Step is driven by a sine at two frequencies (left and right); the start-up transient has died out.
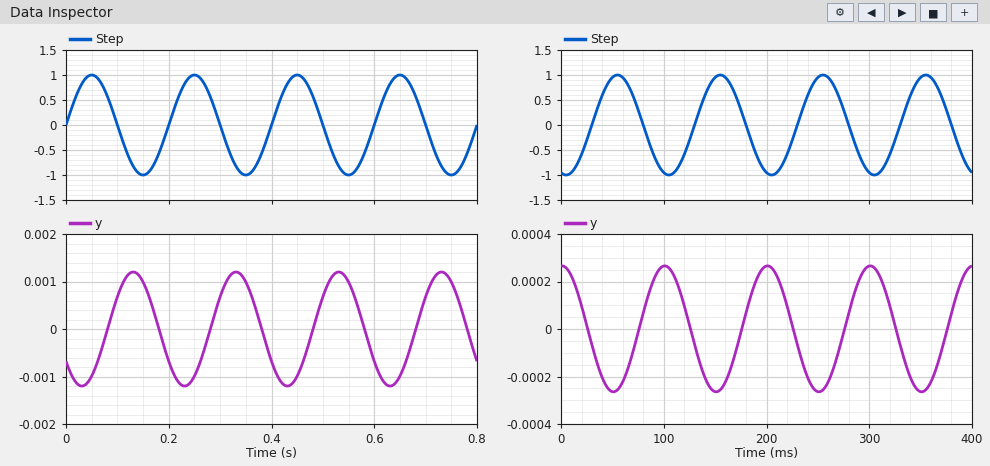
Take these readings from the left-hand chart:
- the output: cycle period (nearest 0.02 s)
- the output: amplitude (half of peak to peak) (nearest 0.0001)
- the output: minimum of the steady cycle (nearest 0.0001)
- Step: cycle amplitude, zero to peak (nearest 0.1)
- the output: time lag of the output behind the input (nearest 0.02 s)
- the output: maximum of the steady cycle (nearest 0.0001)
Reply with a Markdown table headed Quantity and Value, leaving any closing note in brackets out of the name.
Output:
| Quantity | Value |
|---|---|
| the output: cycle period | 0.20 s |
| the output: amplitude (half of peak to peak) | 0.0012 |
| the output: minimum of the steady cycle | -0.0012 |
| Step: cycle amplitude, zero to peak | 1.0 |
| the output: time lag of the output behind the input | 0.08 s |
| the output: maximum of the steady cycle | 0.0012 |
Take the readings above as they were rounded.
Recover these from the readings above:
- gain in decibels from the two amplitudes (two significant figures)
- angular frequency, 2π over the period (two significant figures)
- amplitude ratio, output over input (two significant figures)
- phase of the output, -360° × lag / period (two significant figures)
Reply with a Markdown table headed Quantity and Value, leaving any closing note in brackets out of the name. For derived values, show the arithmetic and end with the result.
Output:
| Quantity | Value |
|---|---|
| gain in decibels from the two amplitudes | 20 log10(0.0012 / 1) = -58 dB |
| angular frequency, 2π over the period | 2π / 0.2 = 31 rad/s |
| amplitude ratio, output over input | 0.0012 / 1 = 0.0012 |
| phase of the output, -360° × lag / period | -360 × 0.08 / 0.2 = -140° |
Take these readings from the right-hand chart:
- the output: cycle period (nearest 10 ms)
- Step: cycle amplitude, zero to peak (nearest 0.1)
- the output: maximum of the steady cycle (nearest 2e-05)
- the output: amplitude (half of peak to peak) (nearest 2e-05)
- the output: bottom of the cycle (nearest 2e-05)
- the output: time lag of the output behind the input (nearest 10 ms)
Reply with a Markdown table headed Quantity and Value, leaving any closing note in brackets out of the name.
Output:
| Quantity | Value |
|---|---|
| the output: cycle period | 100 ms |
| Step: cycle amplitude, zero to peak | 1.0 |
| the output: maximum of the steady cycle | 0.00026 |
| the output: amplitude (half of peak to peak) | 0.00026 |
| the output: bottom of the cycle | -0.00026 |
| the output: time lag of the output behind the input | 50 ms |
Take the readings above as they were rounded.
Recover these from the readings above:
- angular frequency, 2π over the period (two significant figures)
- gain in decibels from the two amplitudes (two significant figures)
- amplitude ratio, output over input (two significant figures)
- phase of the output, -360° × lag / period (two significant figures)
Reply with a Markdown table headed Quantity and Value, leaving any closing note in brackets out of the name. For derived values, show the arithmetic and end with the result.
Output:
| Quantity | Value |
|---|---|
| angular frequency, 2π over the period | 2π / 100 = 0.063 rad/ms |
| gain in decibels from the two amplitudes | 20 log10(0.00026 / 1) = -72 dB |
| amplitude ratio, output over input | 0.00026 / 1 = 0.00026 |
| phase of the output, -360° × lag / period | -360 × 50 / 100 = -180° |
